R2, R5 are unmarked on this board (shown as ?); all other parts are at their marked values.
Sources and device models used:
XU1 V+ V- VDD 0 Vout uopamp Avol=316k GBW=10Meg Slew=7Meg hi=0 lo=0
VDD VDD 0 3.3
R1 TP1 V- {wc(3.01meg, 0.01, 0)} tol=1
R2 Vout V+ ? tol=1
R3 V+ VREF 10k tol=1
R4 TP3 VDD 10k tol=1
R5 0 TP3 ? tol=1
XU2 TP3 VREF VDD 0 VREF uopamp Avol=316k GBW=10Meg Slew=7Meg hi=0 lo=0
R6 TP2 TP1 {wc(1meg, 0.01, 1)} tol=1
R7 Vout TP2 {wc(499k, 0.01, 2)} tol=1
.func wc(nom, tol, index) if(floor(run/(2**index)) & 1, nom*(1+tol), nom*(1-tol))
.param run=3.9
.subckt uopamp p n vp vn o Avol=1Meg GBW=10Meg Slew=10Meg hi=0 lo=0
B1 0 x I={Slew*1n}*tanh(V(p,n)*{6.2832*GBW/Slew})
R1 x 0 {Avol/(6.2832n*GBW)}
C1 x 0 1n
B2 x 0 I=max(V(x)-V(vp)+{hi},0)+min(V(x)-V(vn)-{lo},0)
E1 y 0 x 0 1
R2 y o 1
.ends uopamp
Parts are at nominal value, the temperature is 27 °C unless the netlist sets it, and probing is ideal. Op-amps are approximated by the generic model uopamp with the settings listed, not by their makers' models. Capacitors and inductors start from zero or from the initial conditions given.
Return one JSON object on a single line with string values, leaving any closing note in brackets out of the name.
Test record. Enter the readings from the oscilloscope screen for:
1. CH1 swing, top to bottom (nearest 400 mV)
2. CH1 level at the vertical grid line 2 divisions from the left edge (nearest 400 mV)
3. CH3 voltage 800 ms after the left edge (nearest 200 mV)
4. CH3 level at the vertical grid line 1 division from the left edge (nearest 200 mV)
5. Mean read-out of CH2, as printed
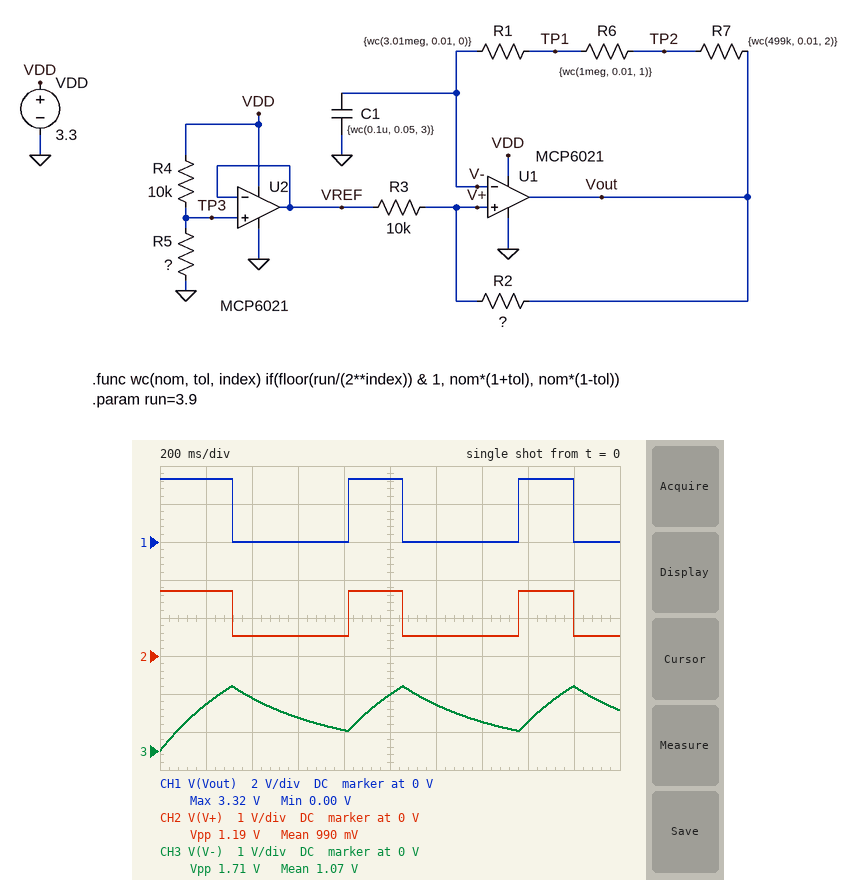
{"CH1 swing, top to bottom": "3.2 V", "CH1 level at the vertical grid line 2 divisions from the left edge": "0 V", "CH3 voltage 800 ms after the left edge": "600 mV", "CH3 level at the vertical grid line 1 division from the left edge": "1.2 V", "Mean read-out of CH2, as printed": "990 mV"}
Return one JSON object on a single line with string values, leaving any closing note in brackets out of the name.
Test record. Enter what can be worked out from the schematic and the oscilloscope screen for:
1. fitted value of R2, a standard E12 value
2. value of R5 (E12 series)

{"fitted value of R2, a standard E12 value": "18 kΩ", "value of R5": "3.3 kΩ"}
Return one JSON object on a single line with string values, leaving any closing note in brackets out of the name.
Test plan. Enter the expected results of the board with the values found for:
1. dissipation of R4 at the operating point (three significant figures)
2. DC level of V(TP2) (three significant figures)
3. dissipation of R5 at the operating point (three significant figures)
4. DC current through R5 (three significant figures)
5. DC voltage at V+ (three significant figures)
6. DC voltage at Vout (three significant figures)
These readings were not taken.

{"dissipation of R4 at the operating point": "616 µW", "DC level of V(TP2)": "819 mV", "dissipation of R5 at the operating point": "203 µW", "DC current through R5": "248 µA", "DC voltage at V+": "819 mV", "DC voltage at Vout": "819 mV"}
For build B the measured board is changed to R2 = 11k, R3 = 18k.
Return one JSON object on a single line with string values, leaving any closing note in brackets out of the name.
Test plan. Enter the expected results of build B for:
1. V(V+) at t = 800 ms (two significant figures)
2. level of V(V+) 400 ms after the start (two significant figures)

{"V(V+) at t = 800 ms": "310 mV", "level of V(V+) 400 ms after the start": "2.4 V"}
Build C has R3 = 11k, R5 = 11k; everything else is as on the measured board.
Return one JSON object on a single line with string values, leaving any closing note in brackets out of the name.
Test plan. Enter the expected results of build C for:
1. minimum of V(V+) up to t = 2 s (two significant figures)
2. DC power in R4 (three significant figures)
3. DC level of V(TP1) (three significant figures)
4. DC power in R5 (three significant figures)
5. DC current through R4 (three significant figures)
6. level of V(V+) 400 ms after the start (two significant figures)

{"minimum of V(V+) up to t = 2 s": "1.1 V", "DC power in R4": "247 µW", "DC level of V(TP1)": "1.73 V", "DC power in R5": "272 µW", "DC current through R4": "157 µA", "level of V(V+) 400 ms after the start": "2.3 V"}
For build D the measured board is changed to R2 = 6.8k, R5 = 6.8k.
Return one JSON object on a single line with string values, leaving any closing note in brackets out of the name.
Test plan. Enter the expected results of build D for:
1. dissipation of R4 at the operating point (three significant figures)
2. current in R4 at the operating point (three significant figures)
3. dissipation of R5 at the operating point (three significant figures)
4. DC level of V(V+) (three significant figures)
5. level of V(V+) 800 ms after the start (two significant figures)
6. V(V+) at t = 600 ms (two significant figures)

{"dissipation of R4 at the operating point": "386 µW", "current in R4 at the operating point": "196 µA", "dissipation of R5 at the operating point": "262 µW", "DC level of V(V+)": "1.34 V", "level of V(V+) 800 ms after the start": "540 mV", "V(V+) at t = 600 ms": "2.5 V"}
